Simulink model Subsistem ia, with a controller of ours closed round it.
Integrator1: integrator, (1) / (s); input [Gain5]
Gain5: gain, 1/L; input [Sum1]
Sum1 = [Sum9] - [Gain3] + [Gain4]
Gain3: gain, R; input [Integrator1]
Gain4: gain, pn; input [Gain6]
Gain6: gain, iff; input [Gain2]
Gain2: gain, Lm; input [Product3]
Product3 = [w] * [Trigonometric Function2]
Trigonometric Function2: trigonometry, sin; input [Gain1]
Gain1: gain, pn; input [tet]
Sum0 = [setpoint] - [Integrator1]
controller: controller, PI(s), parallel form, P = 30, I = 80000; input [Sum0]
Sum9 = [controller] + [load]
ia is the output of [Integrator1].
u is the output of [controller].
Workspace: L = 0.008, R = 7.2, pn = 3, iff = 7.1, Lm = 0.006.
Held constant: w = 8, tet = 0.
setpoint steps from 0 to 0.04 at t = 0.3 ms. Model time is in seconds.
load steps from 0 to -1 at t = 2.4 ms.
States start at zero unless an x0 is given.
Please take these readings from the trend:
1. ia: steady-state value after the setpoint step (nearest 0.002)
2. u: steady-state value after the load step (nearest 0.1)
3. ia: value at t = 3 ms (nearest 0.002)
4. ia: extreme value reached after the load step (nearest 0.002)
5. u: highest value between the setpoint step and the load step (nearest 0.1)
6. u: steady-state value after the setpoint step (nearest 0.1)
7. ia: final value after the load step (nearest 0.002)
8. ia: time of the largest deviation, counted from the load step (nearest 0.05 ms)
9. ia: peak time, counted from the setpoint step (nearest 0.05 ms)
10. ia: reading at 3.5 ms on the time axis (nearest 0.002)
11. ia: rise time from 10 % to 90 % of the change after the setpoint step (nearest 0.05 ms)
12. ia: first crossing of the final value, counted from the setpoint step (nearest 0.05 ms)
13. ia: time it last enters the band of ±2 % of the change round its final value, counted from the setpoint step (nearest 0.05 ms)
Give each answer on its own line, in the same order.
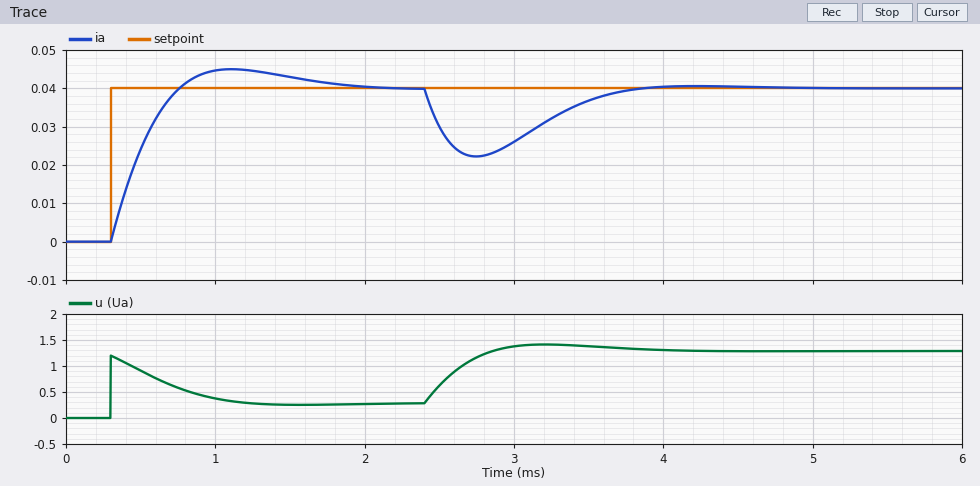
0.040
1.3
0.026
0.022
1.2
0.3
0.040
0.35 ms
0.80 ms
0.036
0.35 ms
0.45 ms
1.60 ms
